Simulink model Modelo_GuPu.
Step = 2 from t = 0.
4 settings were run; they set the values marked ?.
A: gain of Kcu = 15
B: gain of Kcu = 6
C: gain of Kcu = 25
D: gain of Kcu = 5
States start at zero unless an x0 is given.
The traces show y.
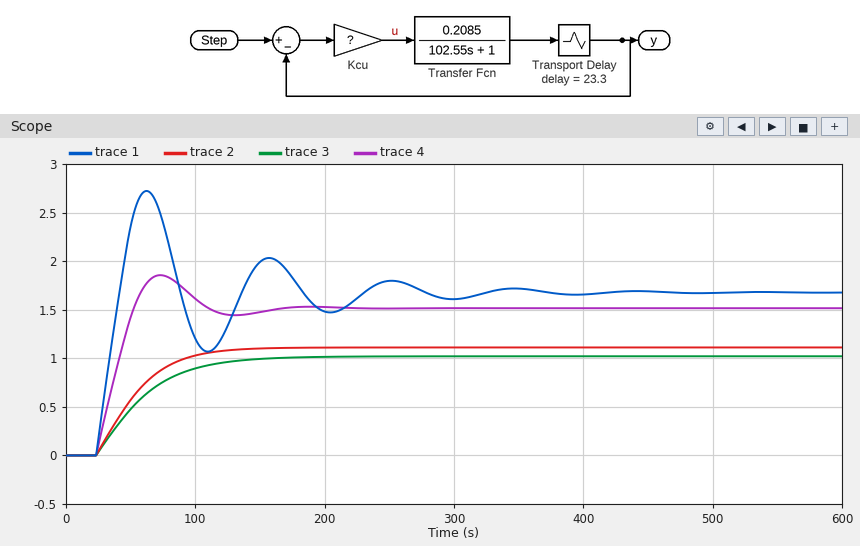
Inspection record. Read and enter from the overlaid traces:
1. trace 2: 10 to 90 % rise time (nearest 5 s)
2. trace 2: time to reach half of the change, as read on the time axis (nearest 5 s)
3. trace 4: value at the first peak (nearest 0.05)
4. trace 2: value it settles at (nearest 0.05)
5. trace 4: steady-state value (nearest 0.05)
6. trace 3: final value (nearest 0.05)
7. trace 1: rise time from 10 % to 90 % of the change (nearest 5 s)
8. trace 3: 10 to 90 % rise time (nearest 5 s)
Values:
65 s
50 s
1.85
1.10
1.50
1.00
15 s
80 s
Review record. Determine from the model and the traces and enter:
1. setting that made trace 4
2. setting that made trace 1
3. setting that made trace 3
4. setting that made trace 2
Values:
A
C
D
B
